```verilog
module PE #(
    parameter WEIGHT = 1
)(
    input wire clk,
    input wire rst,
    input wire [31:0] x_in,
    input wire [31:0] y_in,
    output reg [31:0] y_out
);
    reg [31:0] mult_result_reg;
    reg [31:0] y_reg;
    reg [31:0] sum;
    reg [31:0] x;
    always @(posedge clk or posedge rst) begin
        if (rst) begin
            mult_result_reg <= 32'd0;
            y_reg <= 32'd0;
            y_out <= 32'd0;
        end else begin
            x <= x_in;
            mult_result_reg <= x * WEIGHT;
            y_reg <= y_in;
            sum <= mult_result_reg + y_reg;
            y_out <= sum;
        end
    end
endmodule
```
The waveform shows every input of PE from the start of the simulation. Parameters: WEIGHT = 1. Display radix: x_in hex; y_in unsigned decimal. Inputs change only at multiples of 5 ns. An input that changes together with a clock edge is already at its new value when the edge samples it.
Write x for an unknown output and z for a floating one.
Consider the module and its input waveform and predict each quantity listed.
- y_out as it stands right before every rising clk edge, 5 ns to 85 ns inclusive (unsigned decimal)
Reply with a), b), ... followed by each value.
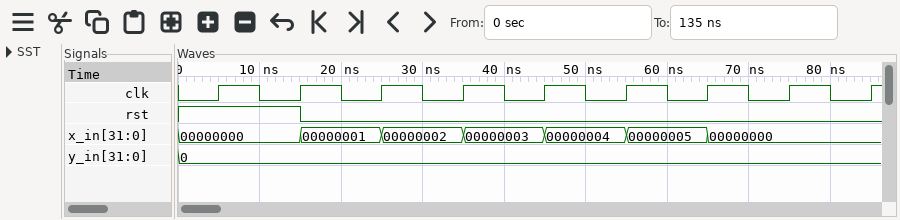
a) 0, 0, x, 0, x, 1, 2, 3, 4
